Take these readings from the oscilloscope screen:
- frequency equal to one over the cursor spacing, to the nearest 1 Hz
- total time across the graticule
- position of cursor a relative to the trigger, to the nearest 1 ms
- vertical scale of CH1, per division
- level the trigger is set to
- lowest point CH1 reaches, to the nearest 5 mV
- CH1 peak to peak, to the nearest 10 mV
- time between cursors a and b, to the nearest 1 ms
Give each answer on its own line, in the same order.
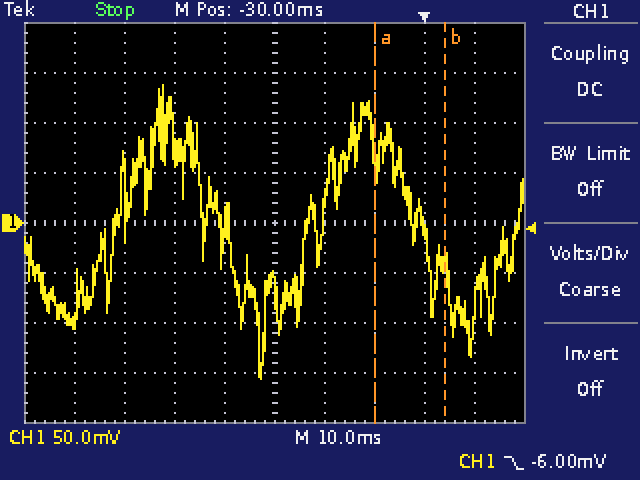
71 Hz
100 ms
-10 ms
50 mV
-6.00 mV
-155 mV
290 mV
14 ms
